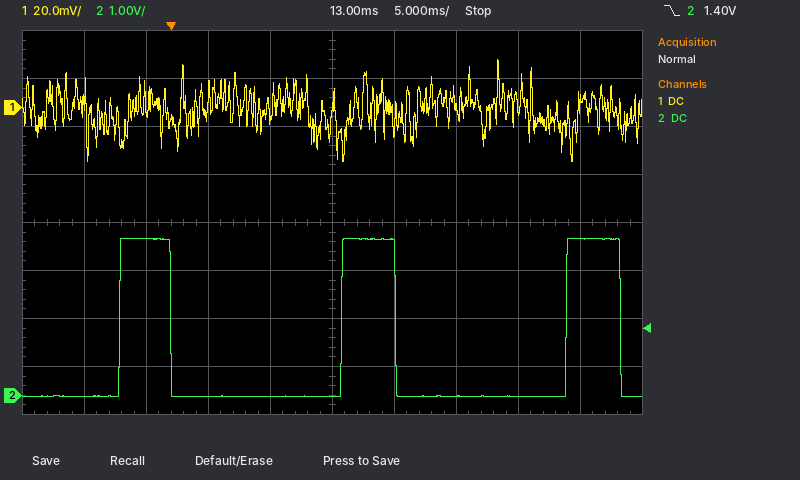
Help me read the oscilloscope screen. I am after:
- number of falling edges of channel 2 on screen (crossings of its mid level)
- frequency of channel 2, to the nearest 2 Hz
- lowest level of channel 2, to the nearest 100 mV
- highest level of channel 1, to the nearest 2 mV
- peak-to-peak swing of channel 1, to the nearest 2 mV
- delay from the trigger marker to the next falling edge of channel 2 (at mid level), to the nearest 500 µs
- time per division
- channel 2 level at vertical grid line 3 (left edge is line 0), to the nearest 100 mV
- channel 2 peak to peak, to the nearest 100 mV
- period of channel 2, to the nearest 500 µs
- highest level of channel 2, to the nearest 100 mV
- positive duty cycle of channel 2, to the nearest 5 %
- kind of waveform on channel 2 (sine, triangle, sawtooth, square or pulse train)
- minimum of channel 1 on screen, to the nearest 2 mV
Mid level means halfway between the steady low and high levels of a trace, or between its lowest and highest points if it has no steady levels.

3
56 Hz
0.0 V
20 mV
42 mV
18.0 ms
5 ms
0.0 V
3.3 V
18.0 ms
3.3 V
25 %
pulse train
-22 mV
